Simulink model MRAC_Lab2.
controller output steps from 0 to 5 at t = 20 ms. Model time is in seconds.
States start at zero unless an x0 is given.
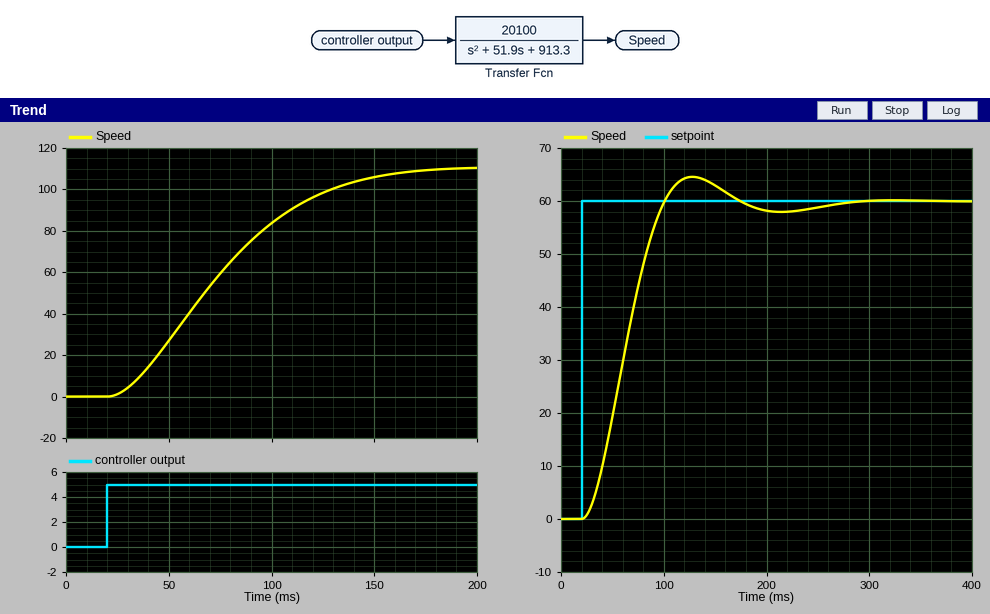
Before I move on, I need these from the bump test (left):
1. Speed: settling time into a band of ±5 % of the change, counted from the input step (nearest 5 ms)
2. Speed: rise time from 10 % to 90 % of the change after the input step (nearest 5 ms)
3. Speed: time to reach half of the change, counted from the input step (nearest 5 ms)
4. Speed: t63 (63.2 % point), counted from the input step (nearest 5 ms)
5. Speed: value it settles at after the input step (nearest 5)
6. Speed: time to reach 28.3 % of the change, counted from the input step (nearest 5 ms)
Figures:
125 ms
90 ms
50 ms
65 ms
110
35 ms
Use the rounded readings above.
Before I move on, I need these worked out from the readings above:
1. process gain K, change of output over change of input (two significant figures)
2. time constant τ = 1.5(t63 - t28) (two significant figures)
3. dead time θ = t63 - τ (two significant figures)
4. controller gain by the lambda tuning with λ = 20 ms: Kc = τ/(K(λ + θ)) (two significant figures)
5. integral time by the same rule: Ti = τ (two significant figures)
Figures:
22
45 ms
20 ms
0.051
45 ms
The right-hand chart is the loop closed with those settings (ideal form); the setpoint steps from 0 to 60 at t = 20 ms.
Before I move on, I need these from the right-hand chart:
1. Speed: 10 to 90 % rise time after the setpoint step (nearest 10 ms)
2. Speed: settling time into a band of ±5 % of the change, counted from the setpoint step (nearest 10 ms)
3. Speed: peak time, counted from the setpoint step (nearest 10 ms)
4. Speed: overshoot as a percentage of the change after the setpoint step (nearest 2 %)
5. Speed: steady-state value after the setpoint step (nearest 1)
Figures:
50 ms
130 ms
110 ms
8 %
60
